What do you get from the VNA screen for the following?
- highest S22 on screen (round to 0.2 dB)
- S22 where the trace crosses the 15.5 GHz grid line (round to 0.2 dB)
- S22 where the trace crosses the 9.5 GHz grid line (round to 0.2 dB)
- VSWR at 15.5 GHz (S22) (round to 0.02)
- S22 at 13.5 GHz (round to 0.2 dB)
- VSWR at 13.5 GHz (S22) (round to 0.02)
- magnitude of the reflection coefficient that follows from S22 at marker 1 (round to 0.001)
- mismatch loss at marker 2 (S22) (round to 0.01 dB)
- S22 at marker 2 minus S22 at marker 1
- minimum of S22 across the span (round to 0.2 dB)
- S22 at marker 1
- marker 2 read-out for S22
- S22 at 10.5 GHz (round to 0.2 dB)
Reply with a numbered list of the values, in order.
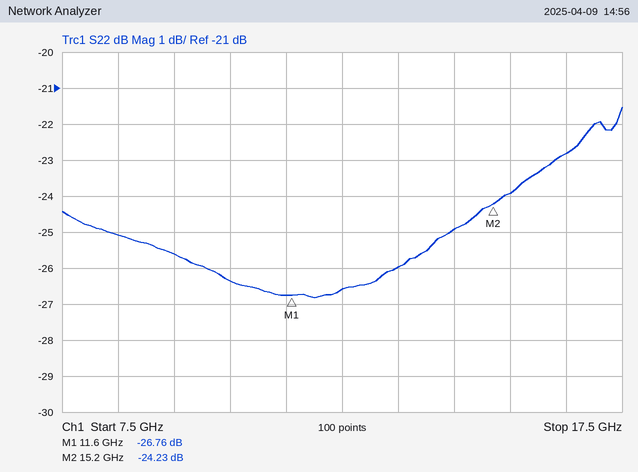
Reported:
1. -21.6 dB
2. -24.0 dB
3. -25.6 dB
4. 1.14
5. -26.0 dB
6. 1.10
7. 0.046
8. 0.02 dB
9. 2.53 dB
10. -26.8 dB
11. -26.76 dB
12. -24.23 dB
13. -26.4 dB
